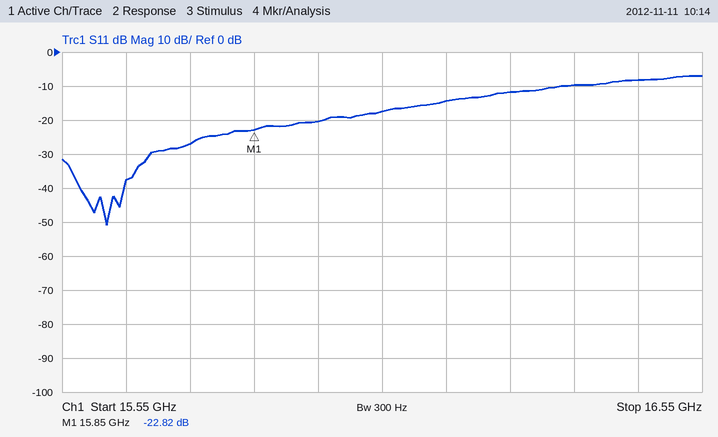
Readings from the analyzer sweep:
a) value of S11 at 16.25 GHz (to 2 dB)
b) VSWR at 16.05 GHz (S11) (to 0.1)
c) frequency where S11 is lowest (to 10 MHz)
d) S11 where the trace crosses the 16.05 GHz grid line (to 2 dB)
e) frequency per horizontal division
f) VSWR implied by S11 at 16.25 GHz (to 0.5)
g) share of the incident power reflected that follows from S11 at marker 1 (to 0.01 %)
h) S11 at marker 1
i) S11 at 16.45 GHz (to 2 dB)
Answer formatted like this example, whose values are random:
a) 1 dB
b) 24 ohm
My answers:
a) -12 dB
b) 1.3
c) 15.62 GHz
d) -18 dB
e) 100 MHz
f) 1.5
g) 0.52 %
h) -22.82 dB
i) -8 dB
